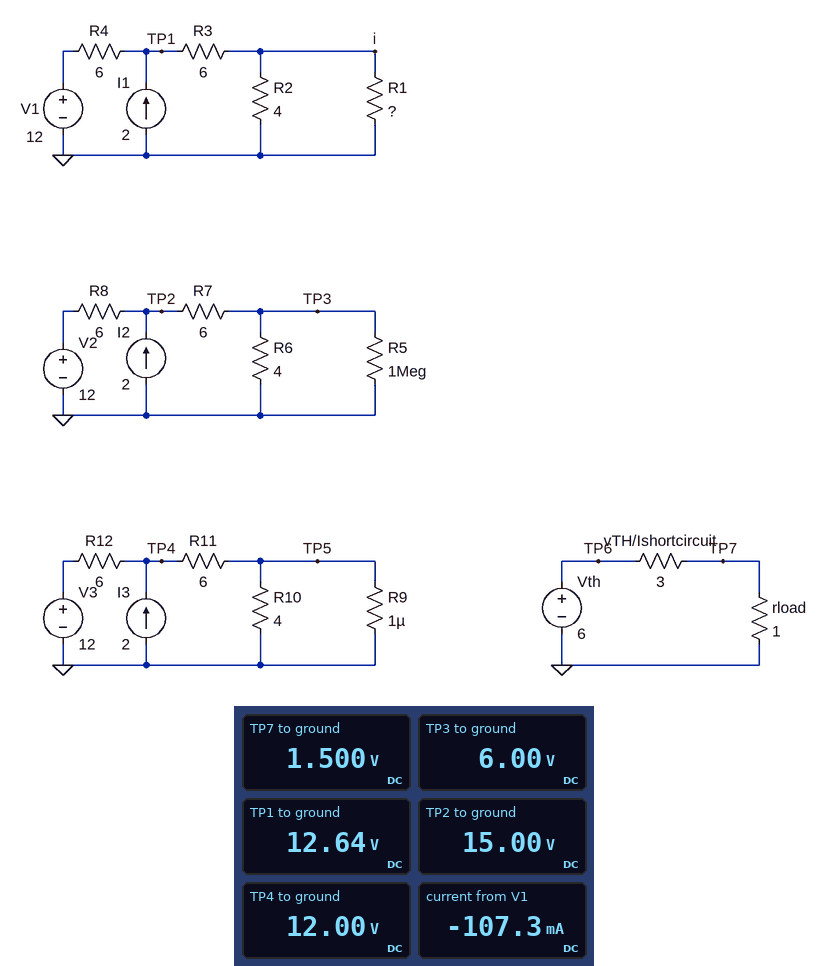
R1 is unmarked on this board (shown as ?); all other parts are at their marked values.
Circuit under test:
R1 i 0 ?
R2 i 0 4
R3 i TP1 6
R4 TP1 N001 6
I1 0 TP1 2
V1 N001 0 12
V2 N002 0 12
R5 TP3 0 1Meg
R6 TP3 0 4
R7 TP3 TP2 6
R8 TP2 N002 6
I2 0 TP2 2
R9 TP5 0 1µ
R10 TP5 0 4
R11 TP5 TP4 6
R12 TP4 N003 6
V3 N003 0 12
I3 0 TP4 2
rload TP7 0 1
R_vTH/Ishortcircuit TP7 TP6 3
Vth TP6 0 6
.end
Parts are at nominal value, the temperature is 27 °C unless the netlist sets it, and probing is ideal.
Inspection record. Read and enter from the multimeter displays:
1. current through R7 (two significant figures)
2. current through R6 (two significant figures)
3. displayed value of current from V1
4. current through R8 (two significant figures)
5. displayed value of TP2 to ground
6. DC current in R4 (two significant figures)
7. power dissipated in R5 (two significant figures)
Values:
1.5 A
1.5 A
-107.3 mA
500 mA
15.00 V
110 mA
36 µW
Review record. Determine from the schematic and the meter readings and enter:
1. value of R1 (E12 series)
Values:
0.82 Ω
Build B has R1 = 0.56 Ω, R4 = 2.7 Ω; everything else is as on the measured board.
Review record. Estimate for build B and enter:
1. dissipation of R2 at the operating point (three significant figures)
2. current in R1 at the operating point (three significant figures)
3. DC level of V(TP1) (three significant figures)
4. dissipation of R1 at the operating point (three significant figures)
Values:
216 mW
1.66 A
12.3 V
1.54 W
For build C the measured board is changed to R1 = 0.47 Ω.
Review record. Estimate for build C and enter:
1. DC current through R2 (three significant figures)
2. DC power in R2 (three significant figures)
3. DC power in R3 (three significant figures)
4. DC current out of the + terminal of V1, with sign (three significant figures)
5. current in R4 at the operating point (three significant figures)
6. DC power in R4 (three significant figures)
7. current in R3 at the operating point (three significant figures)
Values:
203 mA
165 mW
22.4 W
-67.7 mA
67.7 mA
27.5 mW
1.93 A
